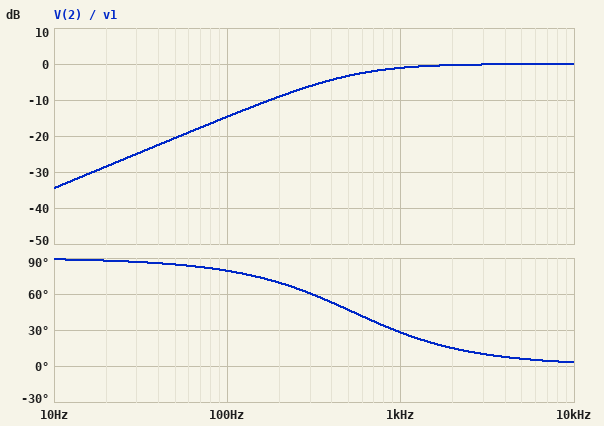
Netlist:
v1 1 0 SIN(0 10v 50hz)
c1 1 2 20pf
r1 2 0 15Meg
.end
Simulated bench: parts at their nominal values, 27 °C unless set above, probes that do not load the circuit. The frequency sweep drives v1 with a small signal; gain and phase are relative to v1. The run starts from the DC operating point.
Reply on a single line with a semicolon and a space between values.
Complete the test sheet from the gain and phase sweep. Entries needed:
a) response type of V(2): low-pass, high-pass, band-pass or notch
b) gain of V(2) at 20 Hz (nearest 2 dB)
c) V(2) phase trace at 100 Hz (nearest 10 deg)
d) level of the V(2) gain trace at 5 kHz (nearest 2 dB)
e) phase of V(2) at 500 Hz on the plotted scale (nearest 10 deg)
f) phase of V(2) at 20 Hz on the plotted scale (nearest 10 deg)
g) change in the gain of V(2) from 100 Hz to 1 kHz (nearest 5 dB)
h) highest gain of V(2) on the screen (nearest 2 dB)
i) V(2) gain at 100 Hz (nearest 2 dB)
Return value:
high-pass; -28 dB; 80 deg; 0 dB; 50 deg; 90 deg; 15 dB; 0 dB; -14 dB
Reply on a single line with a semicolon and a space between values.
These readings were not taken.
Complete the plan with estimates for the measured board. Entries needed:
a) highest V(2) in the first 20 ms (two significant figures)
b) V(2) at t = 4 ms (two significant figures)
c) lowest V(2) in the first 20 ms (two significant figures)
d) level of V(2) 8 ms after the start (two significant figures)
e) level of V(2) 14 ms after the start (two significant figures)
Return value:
930 mV; 370 mV; -940 mV; -700 mV; -370 mV
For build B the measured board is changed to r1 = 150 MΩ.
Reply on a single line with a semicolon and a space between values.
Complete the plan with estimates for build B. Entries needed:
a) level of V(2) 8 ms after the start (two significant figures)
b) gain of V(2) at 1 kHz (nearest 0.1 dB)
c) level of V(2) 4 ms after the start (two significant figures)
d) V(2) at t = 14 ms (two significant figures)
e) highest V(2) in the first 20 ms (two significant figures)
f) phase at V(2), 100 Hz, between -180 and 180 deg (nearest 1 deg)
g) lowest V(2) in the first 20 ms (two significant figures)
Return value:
-1.6 V; 0 dB; 4.7 V; -6.1 V; 5.0 V; 28 deg; -6.9 V
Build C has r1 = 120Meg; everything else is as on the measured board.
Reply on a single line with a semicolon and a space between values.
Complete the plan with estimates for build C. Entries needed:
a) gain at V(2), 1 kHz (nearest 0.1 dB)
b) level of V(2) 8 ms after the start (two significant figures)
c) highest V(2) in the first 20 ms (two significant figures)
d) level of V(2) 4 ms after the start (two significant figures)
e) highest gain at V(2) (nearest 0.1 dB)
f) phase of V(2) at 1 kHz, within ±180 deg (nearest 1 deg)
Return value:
0 dB; -1.9 V; 4.8 V; 4.0 V; 0 dB; 4 deg
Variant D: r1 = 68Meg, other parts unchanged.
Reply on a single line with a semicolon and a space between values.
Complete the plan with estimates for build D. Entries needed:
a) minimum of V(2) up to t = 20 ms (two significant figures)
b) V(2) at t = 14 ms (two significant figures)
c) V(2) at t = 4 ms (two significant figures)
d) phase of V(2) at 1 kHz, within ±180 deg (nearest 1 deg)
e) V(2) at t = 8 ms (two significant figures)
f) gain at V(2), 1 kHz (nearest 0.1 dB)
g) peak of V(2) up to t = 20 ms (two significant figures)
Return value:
-3.9 V; -2.6 V; 2.4 V; 7 deg; -2.0 V; -0.1 dB; 3.6 V
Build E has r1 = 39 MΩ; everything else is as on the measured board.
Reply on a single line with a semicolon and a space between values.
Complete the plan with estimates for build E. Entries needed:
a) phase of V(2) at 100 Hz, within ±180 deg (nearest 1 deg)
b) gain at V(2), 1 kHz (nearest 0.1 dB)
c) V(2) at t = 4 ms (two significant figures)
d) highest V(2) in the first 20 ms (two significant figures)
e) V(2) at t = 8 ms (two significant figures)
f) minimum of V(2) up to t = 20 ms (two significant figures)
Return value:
64 deg; -0.2 dB; 1.2 V; 2.3 V; -1.5 V; -2.4 V
